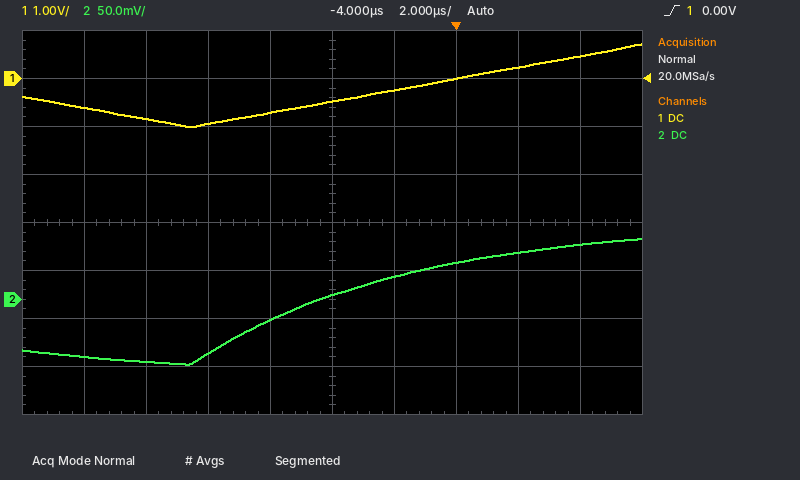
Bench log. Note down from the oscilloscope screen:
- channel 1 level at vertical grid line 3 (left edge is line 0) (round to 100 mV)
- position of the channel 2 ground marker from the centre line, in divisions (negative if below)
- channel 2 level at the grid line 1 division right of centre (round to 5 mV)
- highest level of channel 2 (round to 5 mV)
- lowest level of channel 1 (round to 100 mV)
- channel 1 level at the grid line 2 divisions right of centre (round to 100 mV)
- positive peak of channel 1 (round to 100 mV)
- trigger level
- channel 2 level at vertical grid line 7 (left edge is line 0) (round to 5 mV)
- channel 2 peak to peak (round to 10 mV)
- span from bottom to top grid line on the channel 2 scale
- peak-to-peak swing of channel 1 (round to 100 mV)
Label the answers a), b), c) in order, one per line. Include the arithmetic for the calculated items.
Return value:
a) -900 mV
b) -1.6 div
c) 25 mV
d) 65 mV
e) -1.0 V
f) 0.0 V
g) 700 mV
h) 0.00 V
i) 40 mV
j) 130 mV
k) 400 mV
l) 700 mV − (-1.0 V) = 1.7 V
